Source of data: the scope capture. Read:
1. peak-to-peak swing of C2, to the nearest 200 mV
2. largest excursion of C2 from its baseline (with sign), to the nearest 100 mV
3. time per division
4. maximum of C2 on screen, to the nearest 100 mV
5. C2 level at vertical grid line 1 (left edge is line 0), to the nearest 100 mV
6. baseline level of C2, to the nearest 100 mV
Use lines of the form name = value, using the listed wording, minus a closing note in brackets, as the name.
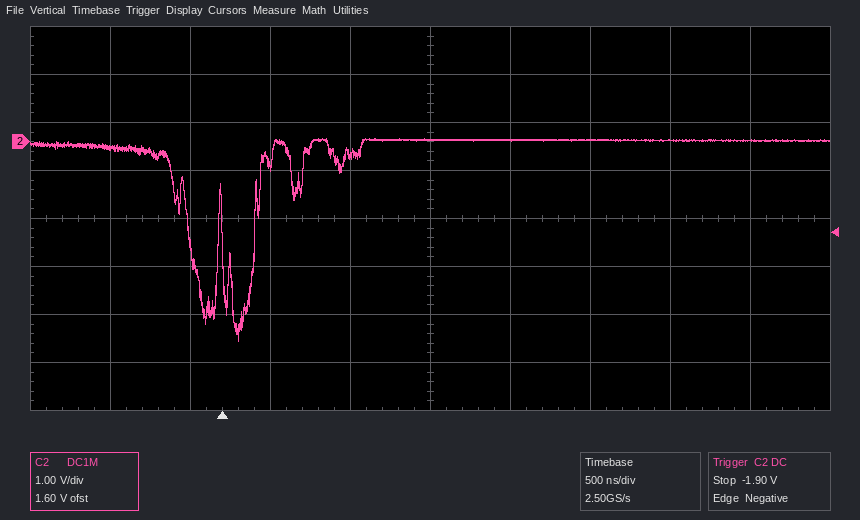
peak-to-peak swing of C2, to the nearest 200 mV = 4.2 V
largest excursion of C2 from its baseline (with sign), to the nearest 100 mV = -4.2 V
time per division = 500 ns
maximum of C2 on screen, to the nearest 100 mV = 100 mV
C2 level at vertical grid line 1 (left edge is line 0), to the nearest 100 mV = -100 mV
baseline level of C2, to the nearest 100 mV = 0.0 V
